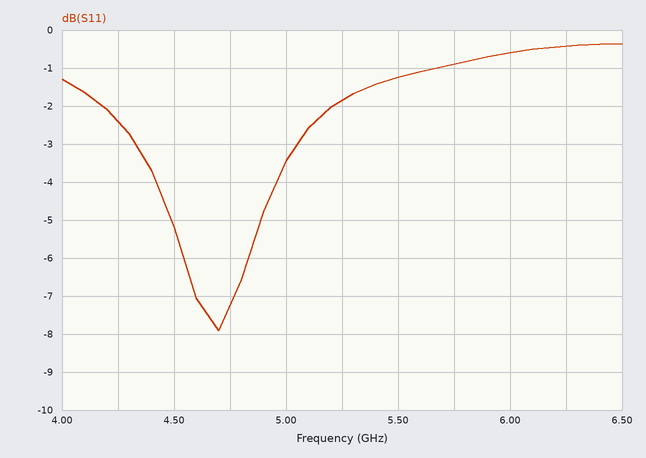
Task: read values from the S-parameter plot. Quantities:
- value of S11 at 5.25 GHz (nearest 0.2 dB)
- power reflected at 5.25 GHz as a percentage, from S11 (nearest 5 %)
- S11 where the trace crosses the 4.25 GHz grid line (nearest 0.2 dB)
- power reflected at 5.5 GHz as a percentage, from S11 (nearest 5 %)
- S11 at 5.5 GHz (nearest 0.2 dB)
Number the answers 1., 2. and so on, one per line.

1. -1.8 dB
2. 65 %
3. -2.4 dB
4. 75 %
5. -1.2 dB
